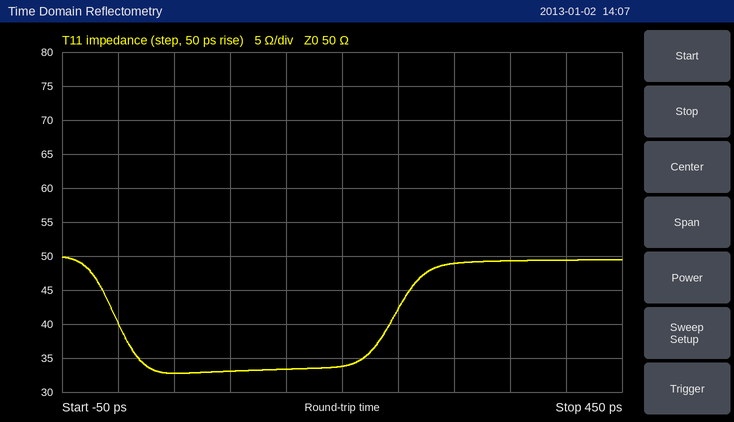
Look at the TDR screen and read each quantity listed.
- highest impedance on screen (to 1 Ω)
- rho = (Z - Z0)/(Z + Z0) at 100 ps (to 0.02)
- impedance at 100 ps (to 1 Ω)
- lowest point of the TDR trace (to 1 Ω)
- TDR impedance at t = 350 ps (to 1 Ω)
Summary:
50 Ω
-0.20
33 Ω
33 Ω
49 Ω
